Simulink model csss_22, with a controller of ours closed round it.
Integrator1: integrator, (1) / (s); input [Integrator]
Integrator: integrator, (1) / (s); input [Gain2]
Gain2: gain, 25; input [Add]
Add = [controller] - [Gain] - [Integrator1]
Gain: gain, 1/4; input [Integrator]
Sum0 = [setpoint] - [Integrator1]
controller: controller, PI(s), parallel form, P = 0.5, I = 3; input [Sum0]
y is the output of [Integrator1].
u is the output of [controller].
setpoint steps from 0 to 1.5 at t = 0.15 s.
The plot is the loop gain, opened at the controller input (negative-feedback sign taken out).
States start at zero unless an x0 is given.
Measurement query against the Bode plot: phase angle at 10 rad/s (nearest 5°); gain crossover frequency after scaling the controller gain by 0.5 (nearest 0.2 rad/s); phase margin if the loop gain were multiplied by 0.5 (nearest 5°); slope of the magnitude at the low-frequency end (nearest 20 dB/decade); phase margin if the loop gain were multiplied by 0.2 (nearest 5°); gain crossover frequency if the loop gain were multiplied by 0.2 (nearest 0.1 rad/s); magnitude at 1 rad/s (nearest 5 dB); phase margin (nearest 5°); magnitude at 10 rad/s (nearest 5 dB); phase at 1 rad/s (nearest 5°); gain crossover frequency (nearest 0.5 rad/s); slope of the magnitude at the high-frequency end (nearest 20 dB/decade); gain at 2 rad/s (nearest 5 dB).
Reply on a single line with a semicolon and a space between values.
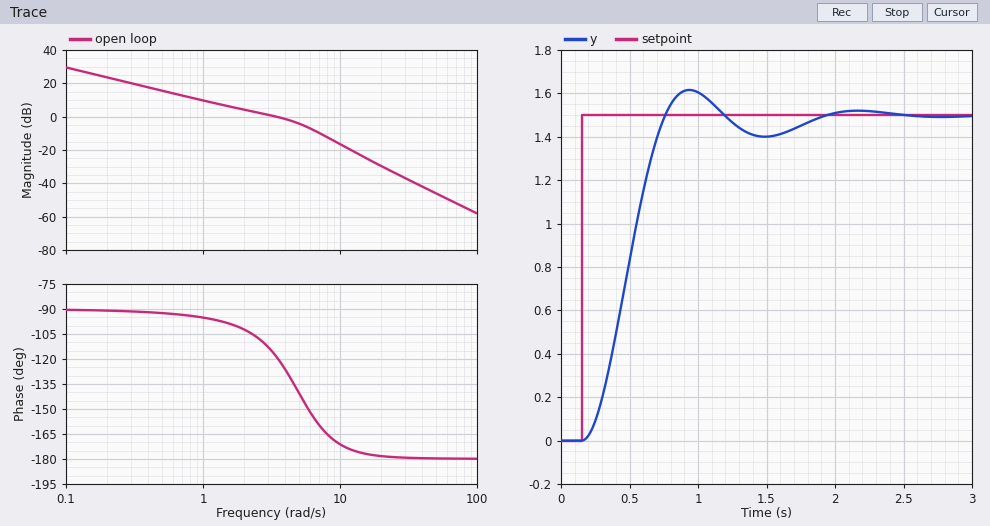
-170°; 1.6 rad/s; 80°; -20 dB/decade; 85°; 0.6 rad/s; 10 dB; 60°; -15 dB; -95°; 3.5 rad/s; -40 dB/decade; 5 dB
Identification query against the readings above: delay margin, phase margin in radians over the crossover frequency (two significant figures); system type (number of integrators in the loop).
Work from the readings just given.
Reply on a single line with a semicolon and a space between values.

0.30 s; 1
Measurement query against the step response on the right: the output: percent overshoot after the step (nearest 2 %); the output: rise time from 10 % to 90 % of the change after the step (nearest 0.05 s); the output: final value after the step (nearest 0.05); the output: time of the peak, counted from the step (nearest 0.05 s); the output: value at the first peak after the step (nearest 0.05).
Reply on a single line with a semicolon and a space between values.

8 %; 0.40 s; 1.50; 0.80 s; 1.60
